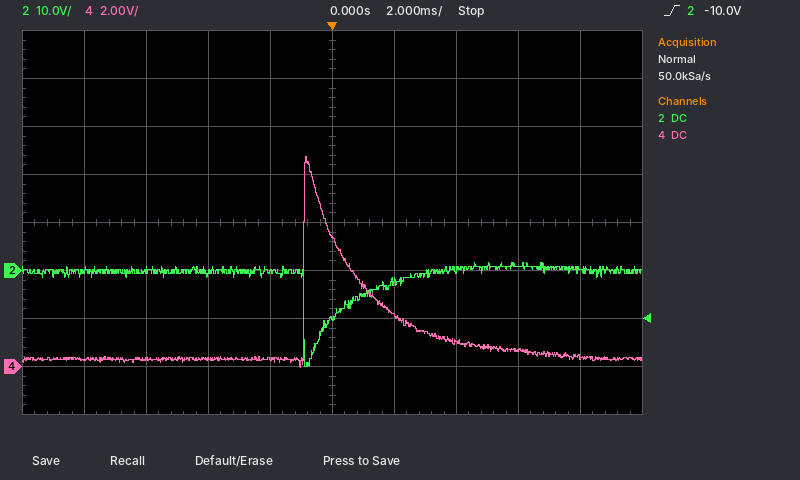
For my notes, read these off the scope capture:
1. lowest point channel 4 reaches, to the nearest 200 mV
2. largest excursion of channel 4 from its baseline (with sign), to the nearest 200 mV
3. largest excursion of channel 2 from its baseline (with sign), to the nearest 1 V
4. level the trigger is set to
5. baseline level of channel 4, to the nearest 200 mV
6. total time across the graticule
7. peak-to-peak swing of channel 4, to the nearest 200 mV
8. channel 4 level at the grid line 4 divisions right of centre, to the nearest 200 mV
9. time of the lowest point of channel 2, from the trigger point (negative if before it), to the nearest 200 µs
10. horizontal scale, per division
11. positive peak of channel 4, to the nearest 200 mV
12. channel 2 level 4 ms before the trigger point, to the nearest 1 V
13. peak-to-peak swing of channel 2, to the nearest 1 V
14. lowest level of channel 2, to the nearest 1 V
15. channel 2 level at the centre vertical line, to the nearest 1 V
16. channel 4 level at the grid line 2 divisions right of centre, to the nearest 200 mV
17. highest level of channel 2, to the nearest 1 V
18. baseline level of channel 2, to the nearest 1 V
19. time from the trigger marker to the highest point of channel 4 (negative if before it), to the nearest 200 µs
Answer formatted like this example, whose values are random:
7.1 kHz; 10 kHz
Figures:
0.0 V; +8.4 V; -20 V; -10.0 V; 400 mV; 20 ms; 8.8 V; 400 mV; -800 µs; 2 ms; 8.8 V; -1 V; 22 V; -20 V; -10 V; 1.0 V; 2 V; 0 V; -800 µs
